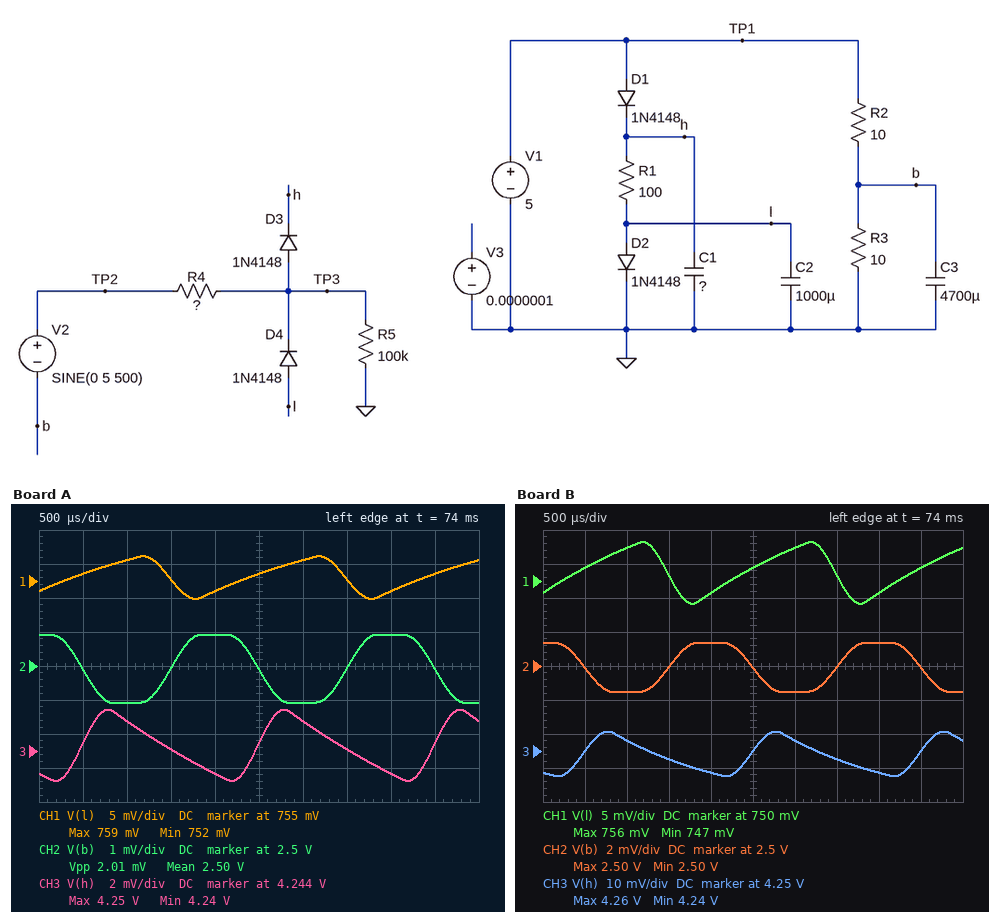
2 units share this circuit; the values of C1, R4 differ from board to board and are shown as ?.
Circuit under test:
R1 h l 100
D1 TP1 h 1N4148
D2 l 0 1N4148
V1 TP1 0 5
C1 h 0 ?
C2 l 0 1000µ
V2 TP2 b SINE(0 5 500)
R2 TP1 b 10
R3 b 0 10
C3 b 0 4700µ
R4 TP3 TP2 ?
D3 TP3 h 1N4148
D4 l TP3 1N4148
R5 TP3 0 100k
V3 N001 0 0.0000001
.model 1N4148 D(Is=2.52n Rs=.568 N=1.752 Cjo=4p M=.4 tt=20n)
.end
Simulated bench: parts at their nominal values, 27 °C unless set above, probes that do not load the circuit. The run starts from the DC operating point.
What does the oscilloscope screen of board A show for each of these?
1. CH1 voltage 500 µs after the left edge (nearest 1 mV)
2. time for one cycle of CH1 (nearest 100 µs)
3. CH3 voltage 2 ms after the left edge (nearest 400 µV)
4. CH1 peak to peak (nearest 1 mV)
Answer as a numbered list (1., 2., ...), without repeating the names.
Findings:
1. 756 mV
2. 2.0 ms
3. 4.2428 V
4. 6 mV
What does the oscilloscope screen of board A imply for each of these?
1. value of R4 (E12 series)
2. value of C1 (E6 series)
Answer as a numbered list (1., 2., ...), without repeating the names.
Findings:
1. 120 Ω
2. 1.5 mF
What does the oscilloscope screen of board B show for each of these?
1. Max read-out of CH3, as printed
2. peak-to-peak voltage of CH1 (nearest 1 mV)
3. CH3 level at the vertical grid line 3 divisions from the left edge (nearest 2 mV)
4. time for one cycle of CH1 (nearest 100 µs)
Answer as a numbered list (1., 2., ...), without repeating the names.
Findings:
1. 4.26 V
2. 9 mV
3. 4.248 V
4. 2.0 ms
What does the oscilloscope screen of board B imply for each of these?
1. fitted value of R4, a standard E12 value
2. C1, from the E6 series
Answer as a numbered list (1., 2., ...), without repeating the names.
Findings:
1. 82 Ω
2. 680 µF
